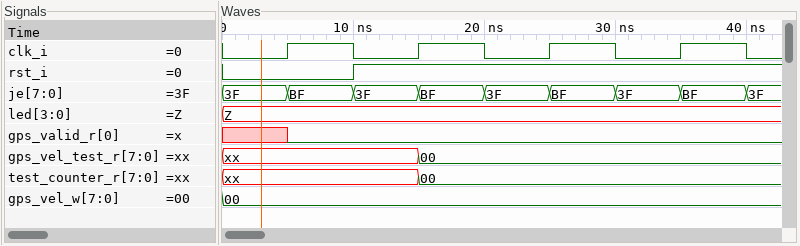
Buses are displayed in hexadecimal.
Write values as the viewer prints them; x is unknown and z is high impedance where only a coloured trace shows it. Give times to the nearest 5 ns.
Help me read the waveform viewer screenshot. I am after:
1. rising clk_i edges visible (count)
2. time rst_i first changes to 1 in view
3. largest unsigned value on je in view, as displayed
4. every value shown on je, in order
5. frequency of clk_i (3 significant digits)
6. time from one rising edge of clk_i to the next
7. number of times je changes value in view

4
10 ns
BF
3F, BF, 3F, BF, 3F, BF, 3F, BF, 3F
100 MHz
10 ns
8
